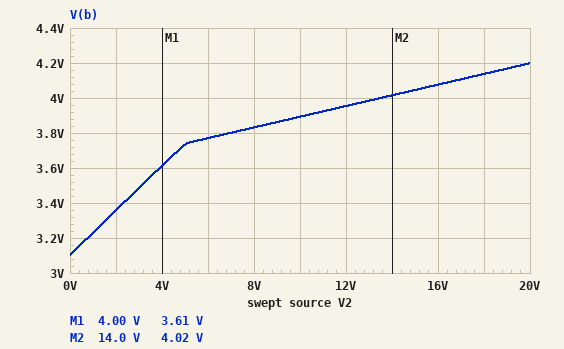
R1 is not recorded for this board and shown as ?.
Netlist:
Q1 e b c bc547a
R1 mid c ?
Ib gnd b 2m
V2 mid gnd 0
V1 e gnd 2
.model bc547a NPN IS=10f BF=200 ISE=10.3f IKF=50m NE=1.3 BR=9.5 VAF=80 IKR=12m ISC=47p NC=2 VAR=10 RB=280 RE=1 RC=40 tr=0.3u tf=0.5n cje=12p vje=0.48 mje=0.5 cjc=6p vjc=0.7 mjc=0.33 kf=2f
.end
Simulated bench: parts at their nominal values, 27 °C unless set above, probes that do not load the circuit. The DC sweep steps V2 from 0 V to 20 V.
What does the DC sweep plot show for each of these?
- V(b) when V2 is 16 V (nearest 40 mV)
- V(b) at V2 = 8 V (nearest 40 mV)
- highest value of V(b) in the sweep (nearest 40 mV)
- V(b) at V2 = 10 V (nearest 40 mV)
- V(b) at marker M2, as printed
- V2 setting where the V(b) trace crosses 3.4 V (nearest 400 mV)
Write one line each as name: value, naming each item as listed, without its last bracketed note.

V(b) when V2 is 16 V: 4.08 V
V(b) at V2 = 8 V: 3.84 V
highest value of V(b) in the sweep: 4.20 V
V(b) at V2 = 10 V: 3.88 V
V(b) at marker M2, as printed: 4.02 V
V2 setting where the V(b) trace crosses 3.4 V: 2.4 V
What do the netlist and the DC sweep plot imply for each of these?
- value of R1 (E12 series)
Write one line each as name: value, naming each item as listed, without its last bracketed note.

value of R1: 270 Ω
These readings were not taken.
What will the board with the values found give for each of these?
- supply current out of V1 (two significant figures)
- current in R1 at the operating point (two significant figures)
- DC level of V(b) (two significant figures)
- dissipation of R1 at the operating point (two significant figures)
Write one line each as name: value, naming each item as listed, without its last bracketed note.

supply current out of V1: 4.6 mA
current in R1 at the operating point: 6.6 mA
DC level of V(b): 3.1 V
dissipation of R1 at the operating point: 12 mW
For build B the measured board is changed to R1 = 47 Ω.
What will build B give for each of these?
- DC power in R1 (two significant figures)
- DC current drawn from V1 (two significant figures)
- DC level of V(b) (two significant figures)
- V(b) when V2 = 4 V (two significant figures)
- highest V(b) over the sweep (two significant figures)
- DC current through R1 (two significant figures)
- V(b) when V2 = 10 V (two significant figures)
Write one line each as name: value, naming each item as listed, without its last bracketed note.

DC power in R1: 25 mW
DC current drawn from V1: 21 mA
DC level of V(b): 2.4 V
V(b) when V2 = 4 V: 3.8 V
highest V(b) over the sweep: 4.4 V
DC current through R1: 23 mA
V(b) when V2 = 10 V: 4.0 V
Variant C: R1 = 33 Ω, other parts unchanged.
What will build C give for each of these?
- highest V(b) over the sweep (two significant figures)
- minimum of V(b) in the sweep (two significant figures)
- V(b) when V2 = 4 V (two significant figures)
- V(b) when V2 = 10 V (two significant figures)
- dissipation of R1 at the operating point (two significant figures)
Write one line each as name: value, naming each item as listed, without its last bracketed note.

highest V(b) over the sweep: 4.4 V
minimum of V(b) in the sweep: 2.3 V
V(b) when V2 = 4 V: 3.8 V
V(b) when V2 = 10 V: 4.0 V
dissipation of R1 at the operating point: 25 mW
